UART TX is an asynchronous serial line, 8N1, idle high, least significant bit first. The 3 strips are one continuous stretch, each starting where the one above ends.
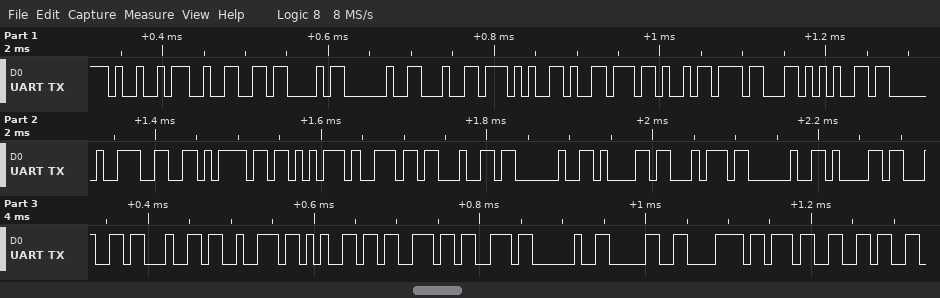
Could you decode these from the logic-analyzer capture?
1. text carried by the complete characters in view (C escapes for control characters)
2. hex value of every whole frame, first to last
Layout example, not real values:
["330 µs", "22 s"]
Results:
["\"I2C device found at address 0x76\"", "49 32 43 20 64 65 76 69 63 65 20 66 6F 75 6E 64 20 61 74 20 61 64 64 72 65 73 73 20 30 78 37 36"]
